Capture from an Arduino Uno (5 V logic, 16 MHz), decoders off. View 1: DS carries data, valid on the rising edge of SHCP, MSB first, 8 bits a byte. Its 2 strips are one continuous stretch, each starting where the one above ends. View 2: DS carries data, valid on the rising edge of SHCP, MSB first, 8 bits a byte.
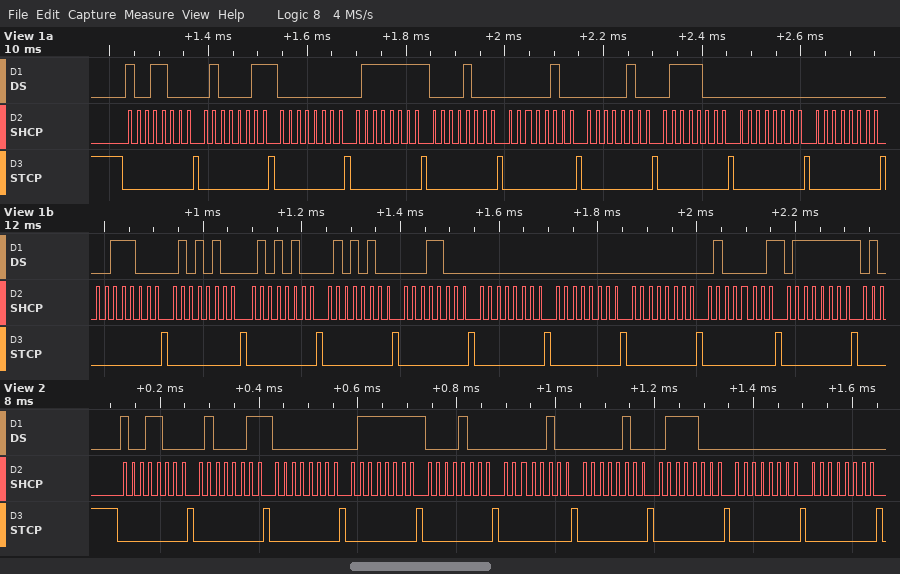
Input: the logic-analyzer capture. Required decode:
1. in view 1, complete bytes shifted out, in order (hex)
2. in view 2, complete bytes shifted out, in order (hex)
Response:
98 43 00 7F 08 04 04 78 00 00 38 54 54 54 18 00 00 00 41 7F
98 43 00 7F 08 04 04 78 00 00
